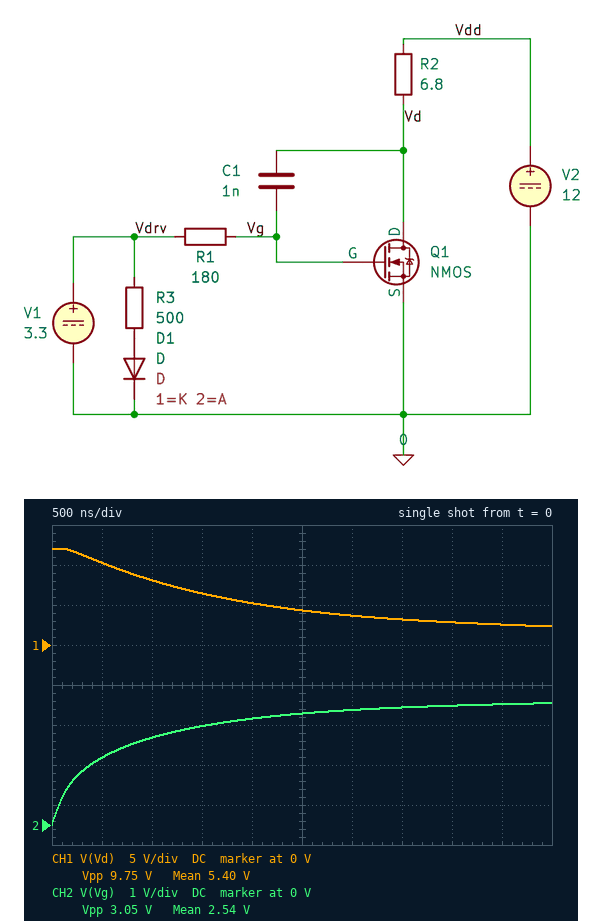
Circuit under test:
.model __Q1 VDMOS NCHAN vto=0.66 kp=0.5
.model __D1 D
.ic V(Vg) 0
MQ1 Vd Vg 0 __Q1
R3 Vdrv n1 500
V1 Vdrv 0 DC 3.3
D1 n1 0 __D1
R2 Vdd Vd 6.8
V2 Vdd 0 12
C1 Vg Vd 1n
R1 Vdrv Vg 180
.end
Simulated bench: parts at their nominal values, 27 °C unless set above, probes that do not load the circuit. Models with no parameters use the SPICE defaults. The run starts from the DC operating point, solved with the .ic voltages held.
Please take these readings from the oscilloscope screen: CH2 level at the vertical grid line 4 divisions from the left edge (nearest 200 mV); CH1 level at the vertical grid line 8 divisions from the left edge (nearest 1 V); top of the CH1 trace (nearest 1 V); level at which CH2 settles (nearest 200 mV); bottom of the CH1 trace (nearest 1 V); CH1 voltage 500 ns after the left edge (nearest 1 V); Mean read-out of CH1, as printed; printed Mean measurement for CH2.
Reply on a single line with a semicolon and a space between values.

2.6 V; 3 V; 12 V; 3.0 V; 2 V; 10 V; 5.40 V; 2.54 V
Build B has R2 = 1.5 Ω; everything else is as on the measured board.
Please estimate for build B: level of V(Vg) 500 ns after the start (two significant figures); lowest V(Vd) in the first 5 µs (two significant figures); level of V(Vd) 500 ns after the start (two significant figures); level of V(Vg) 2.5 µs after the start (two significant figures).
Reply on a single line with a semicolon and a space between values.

2.0 V; 9.4 V; 11 V; 3.2 V
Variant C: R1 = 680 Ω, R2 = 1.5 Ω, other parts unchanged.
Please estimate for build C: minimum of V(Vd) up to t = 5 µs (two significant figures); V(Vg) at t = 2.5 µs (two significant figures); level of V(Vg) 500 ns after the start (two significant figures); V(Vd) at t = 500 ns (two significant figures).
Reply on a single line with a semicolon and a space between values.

10 V; 2.3 V; 840 mV; 12 V
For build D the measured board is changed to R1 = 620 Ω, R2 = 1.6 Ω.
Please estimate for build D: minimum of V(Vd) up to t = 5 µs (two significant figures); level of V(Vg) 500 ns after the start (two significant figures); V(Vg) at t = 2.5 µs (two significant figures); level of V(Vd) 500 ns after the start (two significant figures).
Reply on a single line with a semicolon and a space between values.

9.9 V; 900 mV; 2.4 V; 12 V
